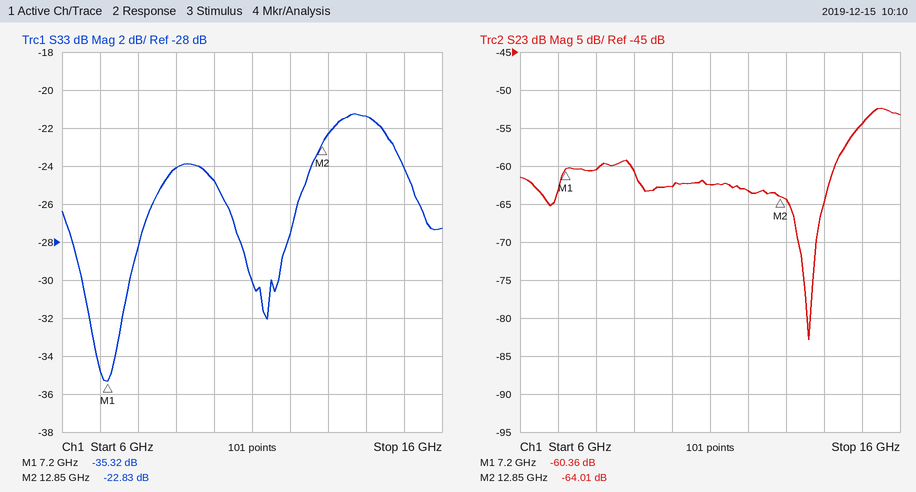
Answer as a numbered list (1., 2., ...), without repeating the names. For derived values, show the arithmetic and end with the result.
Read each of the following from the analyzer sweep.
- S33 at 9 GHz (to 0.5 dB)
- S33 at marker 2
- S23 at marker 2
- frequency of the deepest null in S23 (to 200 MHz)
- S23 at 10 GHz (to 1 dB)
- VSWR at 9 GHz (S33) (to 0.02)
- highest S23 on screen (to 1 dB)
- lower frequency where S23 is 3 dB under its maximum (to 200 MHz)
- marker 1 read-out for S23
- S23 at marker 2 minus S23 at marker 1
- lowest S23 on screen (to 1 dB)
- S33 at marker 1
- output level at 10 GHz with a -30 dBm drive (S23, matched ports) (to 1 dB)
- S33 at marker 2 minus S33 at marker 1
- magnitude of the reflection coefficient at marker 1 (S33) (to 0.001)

1. -24.0 dB
2. -22.83 dB
3. -64.01 dB
4. 13.6 GHz
5. -63 dB
6. |Γ| = 10^(-24/20) = 0.0631; VSWR = (1 + 0.0631)/(1 − 0.0631) ≈ 1.13, so 1.14 to the nearest 0.02
7. -52 dB
8. 14.8 GHz
9. -60.36 dB
10. -64.01 − (-60.36) = -3.65 dB
11. -83 dB
12. -35.32 dB
13. -30 dBm + (-63 dB) = -93 dBm
14. -22.83 − (-35.32) = 12.49 dB
15. 10^(-35.32/20) ≈ 0.017
